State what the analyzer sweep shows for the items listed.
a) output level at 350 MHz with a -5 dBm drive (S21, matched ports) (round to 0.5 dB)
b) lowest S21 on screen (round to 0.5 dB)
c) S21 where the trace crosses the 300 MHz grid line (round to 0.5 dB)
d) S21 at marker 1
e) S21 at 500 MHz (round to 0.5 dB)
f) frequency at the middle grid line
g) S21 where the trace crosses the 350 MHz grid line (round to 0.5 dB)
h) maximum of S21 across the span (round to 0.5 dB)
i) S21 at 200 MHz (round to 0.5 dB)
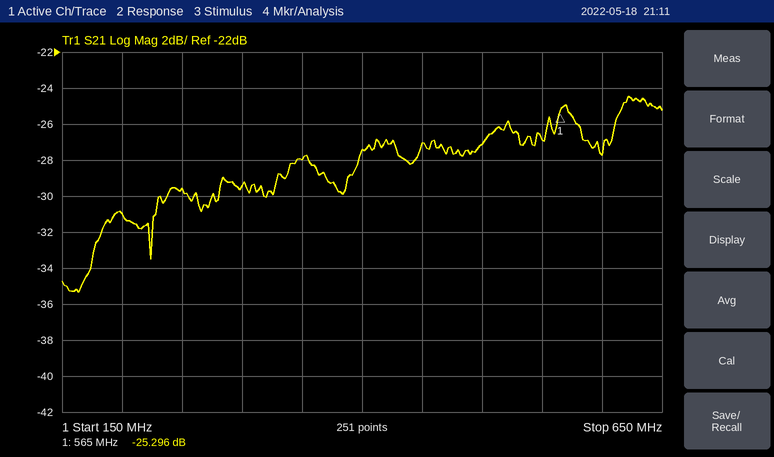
-33.0 dBm
-35.5 dB
-29.5 dB
-25.296 dB
-27.0 dB
400 MHz
-28.0 dB
-24.5 dB
-31.0 dB
